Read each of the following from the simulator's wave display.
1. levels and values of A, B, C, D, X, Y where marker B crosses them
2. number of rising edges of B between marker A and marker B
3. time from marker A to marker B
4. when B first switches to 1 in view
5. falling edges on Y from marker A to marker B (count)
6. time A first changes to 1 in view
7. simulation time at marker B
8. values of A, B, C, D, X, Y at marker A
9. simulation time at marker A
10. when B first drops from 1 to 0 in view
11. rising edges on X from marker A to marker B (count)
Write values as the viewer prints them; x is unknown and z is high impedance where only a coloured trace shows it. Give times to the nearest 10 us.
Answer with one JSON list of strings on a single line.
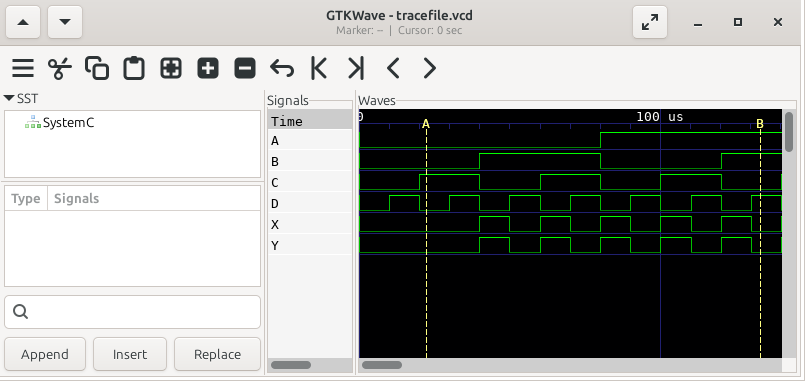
["A=1, B=1, C=0, D=1, X=0, Y=0", "2", "110 us", "40 us", "5", "80 us", "130 us", "A=0, B=0, C=1, D=0, X=0, Y=0", "20 us", "80 us", "5"]
